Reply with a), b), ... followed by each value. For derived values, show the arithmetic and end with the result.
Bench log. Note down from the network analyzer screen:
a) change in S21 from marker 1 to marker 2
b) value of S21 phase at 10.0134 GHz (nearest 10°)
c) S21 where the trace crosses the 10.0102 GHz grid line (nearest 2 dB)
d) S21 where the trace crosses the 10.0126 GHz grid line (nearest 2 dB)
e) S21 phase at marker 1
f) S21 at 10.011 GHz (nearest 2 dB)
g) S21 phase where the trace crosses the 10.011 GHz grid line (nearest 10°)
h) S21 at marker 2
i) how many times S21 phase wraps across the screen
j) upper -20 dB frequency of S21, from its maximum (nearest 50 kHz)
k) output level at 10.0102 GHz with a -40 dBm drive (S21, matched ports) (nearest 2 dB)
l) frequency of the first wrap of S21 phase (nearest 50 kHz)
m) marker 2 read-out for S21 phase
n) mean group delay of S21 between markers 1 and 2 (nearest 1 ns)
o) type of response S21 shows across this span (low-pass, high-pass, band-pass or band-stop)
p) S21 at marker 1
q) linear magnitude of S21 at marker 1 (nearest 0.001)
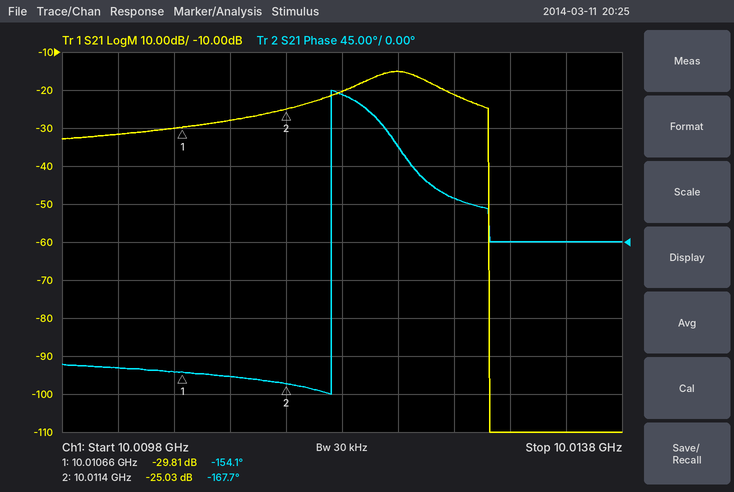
a) -25.03 − (-29.81) = 4.78 dB
b) 0°
c) -32 dB
d) -22 dB
e) -154.1°
f) -28 dB
g) -160°
h) -25.03 dB
i) 1
j) 10.01285 GHz
k) -40 dBm + (-32 dB) = -72 dBm
l) 10.01170 GHz
m) -167.7°
n) −(-167.7° − (-154.1°))/(360° × 740 kHz) ≈ 51 ns
o) band-pass
p) -29.81 dB
q) 10^(-29.81/20) ≈ 0.032
